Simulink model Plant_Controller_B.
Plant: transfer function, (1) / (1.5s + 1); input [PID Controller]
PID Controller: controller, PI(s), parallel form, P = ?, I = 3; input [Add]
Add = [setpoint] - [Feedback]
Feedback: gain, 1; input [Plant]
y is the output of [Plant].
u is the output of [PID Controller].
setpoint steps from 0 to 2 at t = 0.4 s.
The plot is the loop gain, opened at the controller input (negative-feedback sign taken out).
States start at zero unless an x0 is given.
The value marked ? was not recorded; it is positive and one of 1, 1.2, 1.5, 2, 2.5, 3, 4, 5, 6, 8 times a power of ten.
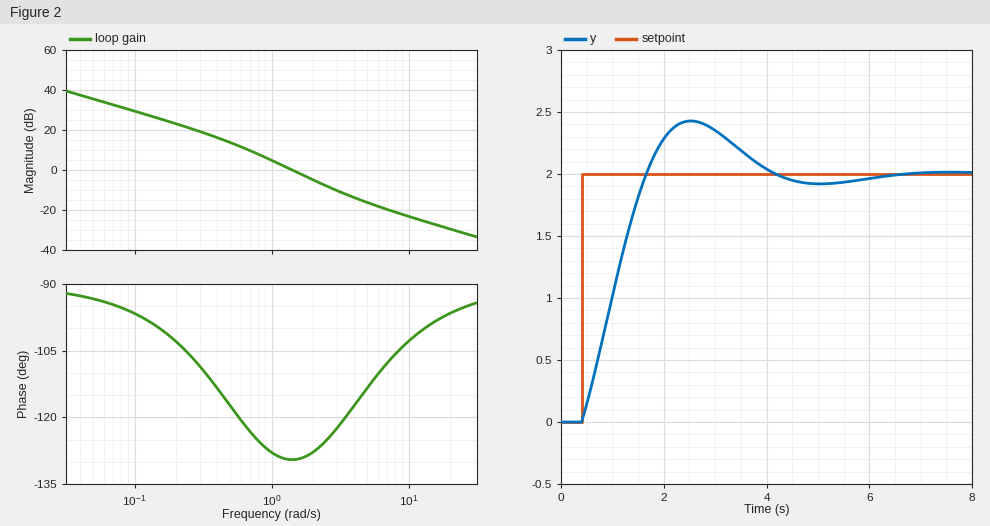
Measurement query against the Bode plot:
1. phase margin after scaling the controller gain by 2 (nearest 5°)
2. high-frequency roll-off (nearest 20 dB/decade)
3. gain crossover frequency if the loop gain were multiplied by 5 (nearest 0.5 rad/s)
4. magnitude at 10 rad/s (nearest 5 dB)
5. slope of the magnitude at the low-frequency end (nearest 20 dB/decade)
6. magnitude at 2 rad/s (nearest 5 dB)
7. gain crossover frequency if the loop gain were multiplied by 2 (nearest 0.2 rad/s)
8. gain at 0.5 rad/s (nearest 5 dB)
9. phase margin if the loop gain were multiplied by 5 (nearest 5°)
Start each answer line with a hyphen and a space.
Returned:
- 55°
- -20 dB/decade
- 4.0 rad/s
- -25 dB
- -20 dB/decade
- -5 dB
- 2.2 rad/s
- 15 dB
- 65°
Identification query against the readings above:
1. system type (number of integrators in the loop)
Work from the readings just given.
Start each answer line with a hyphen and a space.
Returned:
- 1
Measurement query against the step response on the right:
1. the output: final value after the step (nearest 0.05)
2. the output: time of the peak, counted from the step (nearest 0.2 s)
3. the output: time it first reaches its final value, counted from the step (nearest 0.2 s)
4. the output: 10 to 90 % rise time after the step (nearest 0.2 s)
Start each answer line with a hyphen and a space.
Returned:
- 2.00
- 2.2 s
- 1.2 s
- 1.0 s
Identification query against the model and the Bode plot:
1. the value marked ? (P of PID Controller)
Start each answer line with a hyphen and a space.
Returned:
- 1
